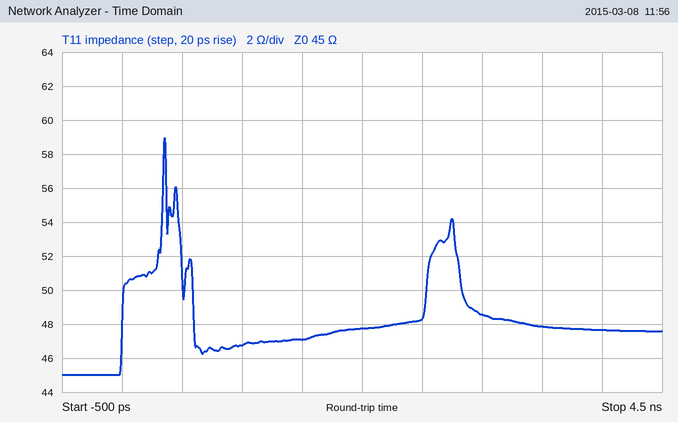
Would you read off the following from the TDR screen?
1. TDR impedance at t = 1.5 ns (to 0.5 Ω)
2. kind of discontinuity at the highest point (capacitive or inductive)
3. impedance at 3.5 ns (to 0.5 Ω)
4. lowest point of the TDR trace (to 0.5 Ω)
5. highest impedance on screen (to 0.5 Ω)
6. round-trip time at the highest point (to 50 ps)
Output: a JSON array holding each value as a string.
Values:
["47.0 Ω", "inductive", "48.0 Ω", "45.0 Ω", "59.0 Ω", "350 ps"]
